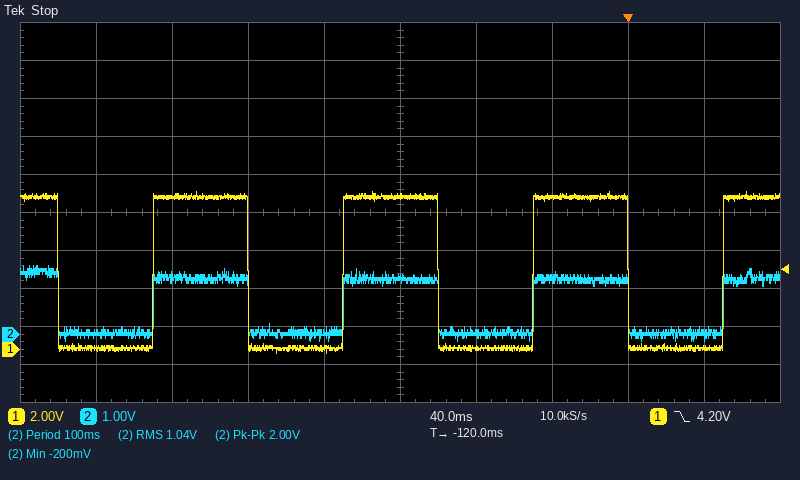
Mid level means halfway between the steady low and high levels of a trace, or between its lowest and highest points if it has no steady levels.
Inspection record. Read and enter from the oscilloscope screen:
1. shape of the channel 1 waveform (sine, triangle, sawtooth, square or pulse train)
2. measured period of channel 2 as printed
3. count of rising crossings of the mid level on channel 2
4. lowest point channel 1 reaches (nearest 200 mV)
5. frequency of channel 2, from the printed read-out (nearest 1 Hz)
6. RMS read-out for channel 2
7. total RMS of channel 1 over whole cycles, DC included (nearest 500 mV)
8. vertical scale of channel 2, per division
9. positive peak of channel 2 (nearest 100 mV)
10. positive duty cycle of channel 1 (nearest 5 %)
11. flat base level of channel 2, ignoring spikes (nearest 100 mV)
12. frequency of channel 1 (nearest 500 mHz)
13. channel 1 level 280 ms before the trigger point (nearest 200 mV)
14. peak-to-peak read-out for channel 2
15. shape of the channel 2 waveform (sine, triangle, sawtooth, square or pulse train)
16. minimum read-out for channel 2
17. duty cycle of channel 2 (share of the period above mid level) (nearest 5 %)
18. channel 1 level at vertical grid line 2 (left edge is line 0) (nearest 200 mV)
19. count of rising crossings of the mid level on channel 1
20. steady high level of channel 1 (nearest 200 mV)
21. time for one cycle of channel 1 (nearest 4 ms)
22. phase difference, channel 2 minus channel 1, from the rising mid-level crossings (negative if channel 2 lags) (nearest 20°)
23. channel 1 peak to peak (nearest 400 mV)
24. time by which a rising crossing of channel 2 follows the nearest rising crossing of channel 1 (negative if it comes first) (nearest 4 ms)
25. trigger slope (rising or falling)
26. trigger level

square
100 ms
4
-200 mV
10 Hz
1.04 V
5.5 V
1 V
1.8 V
50 %
0.0 V
10.0 Hz
0.0 V
2.00 V
square
-200 mV
50 %
8.0 V
4
8.0 V
100 ms
0°
8.4 V
0 ms
falling
4.20 V
